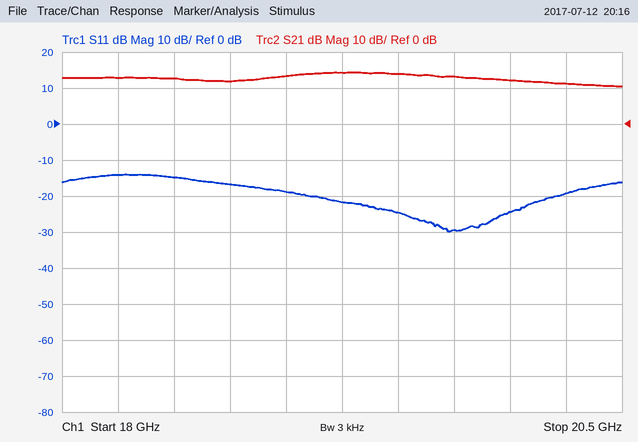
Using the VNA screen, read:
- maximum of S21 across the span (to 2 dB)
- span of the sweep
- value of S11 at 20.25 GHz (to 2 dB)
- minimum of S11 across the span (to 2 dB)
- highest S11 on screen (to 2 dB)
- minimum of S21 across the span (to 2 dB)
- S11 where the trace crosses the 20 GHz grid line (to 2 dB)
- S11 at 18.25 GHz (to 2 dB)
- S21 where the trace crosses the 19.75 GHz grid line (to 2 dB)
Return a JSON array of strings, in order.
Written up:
["14 dB", "2.5 GHz", "-20 dB", "-30 dB", "-14 dB", "10 dB", "-24 dB", "-14 dB", "14 dB"]
